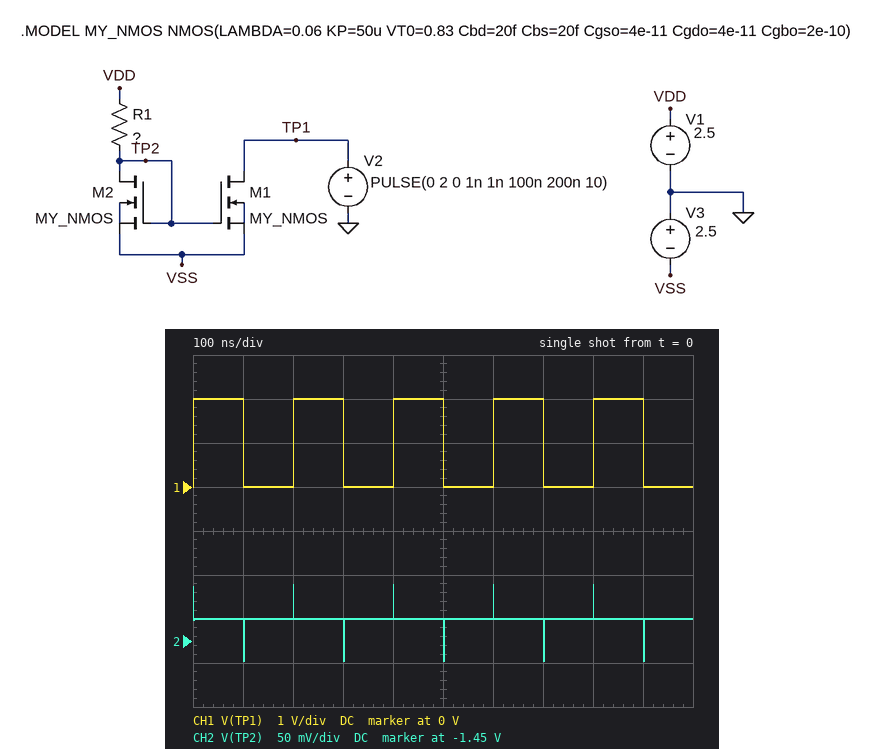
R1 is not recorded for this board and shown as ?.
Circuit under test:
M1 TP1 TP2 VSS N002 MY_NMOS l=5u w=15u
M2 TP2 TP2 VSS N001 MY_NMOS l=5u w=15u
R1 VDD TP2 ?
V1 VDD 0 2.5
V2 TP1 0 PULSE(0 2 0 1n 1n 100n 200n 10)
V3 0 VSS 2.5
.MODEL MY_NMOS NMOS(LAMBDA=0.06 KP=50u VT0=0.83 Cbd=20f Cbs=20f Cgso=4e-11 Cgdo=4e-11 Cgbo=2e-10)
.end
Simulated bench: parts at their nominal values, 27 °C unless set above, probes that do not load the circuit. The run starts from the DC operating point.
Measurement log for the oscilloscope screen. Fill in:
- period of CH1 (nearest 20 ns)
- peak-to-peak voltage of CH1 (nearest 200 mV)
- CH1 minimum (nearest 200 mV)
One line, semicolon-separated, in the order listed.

200 ns; 2.0 V; 0 V
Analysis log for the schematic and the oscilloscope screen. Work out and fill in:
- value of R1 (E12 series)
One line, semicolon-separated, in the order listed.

820 kΩ
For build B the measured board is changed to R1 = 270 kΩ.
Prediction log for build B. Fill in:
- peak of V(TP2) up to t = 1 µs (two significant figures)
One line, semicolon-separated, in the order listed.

-1.2 V
